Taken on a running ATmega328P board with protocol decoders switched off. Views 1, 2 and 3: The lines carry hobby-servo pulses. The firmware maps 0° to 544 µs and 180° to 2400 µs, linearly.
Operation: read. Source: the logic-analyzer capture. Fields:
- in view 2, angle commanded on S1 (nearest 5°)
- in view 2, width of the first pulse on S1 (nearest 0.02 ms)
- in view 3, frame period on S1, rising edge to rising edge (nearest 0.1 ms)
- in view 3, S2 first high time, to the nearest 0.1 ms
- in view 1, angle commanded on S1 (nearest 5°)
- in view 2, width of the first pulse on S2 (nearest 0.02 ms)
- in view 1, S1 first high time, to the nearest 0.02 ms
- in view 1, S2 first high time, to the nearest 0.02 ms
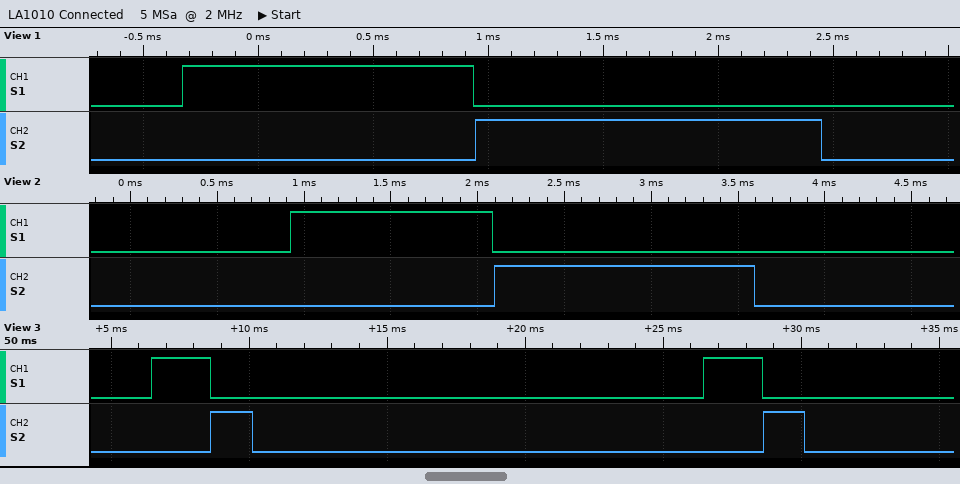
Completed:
60°
1.16 ms
20.0 ms
1.5 ms
70°
1.50 ms
1.26 ms
1.50 ms
